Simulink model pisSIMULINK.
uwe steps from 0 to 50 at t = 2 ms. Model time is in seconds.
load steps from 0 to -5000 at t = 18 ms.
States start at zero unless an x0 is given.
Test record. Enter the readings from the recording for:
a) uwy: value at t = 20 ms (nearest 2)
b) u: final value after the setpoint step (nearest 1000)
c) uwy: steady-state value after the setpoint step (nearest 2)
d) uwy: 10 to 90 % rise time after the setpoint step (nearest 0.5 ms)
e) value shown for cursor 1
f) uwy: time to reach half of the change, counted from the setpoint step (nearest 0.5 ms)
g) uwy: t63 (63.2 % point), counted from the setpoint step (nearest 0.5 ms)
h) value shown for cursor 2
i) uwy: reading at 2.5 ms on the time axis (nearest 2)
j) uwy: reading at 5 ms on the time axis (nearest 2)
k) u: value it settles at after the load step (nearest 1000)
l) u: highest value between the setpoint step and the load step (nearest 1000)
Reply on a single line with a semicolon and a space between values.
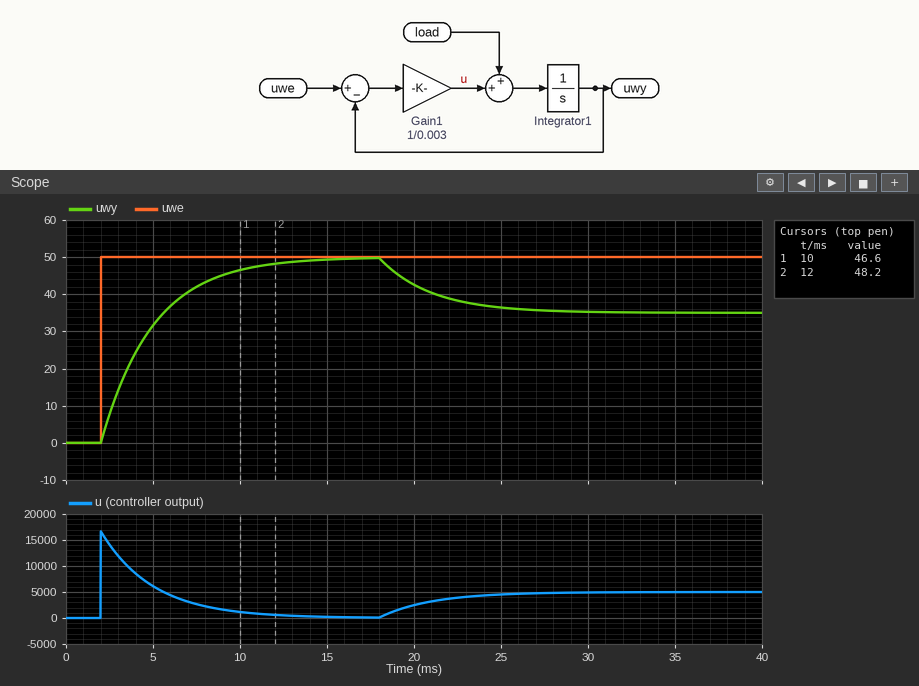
42; 0; 50; 6.5 ms; 46.6; 2.0 ms; 3.0 ms; 48.2; 8; 32; 5000; 17000
